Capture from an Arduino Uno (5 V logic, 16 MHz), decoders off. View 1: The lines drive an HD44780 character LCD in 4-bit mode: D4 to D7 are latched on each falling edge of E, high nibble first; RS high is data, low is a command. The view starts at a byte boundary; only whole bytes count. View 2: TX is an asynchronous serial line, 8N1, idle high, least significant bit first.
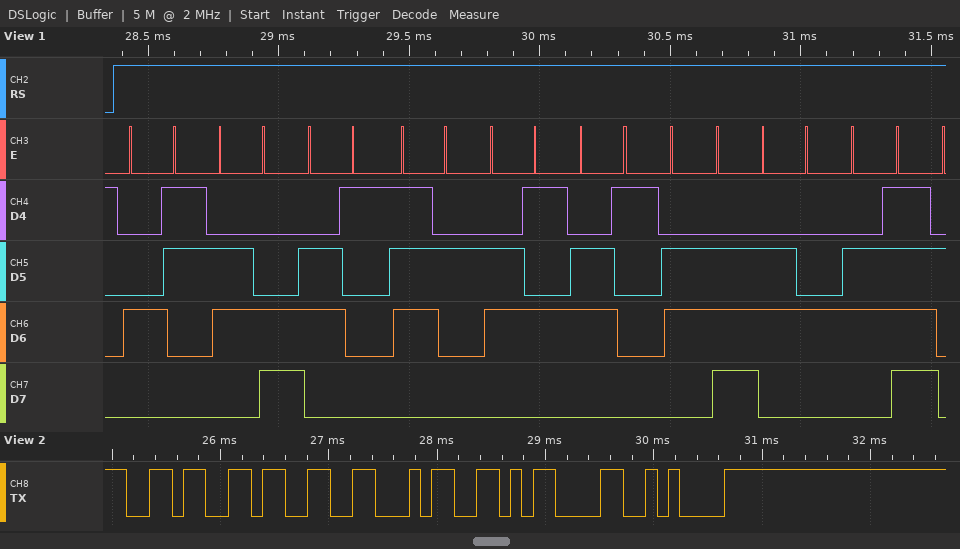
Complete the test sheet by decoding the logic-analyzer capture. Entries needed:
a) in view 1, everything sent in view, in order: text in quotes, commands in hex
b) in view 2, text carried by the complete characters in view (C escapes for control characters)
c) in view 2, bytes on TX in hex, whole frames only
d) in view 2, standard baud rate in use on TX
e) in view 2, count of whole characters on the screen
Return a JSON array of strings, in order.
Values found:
["\"Clareando\"", "\"634\\r\\n\"", "36 33 34 0D 0A", "9600 baud", "5"]
